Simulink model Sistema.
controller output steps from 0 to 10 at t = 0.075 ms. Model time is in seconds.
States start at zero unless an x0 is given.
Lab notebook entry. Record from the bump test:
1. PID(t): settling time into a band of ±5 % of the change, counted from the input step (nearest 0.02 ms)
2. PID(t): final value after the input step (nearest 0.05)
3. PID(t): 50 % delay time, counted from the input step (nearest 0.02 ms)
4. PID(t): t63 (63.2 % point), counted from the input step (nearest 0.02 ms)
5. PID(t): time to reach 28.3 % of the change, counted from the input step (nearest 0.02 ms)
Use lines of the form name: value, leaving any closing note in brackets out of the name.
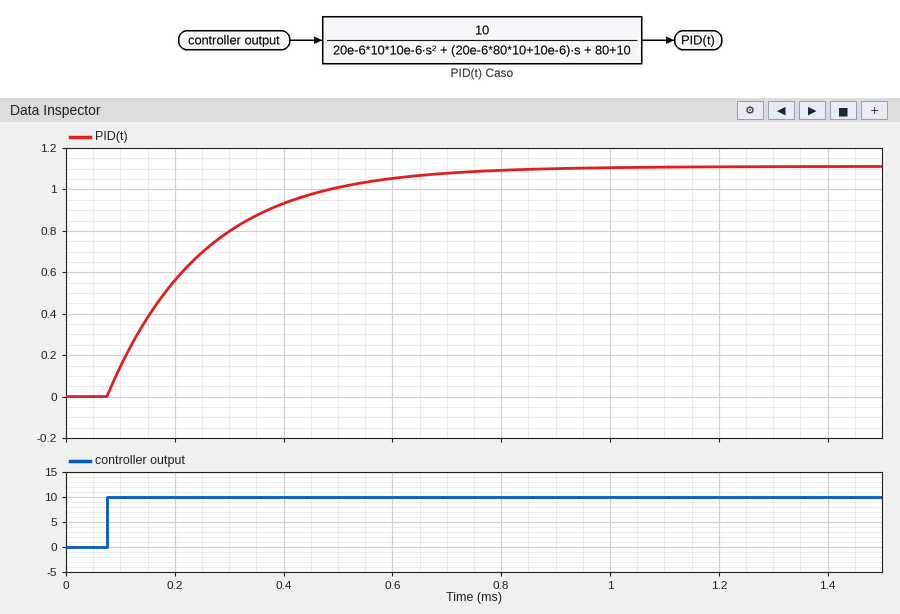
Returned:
PID(t): settling time into a band of ±5 % of the change, counted from the input step: 0.54 ms
PID(t): final value after the input step: 1.10
PID(t): 50 % delay time, counted from the input step: 0.12 ms
PID(t): t63 (63.2 % point), counted from the input step: 0.18 ms
PID(t): time to reach 28.3 % of the change, counted from the input step: 0.06 ms
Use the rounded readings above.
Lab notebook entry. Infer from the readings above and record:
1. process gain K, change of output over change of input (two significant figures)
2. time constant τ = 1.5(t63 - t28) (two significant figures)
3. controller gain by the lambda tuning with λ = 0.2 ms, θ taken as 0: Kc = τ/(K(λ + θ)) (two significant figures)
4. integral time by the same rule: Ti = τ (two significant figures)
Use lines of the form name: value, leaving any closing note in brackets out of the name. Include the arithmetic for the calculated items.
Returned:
process gain K, change of output over change of input: (1.1 - 0) / 10 = 0.11
time constant τ = 1.5(t63 - t28): 1.5 × (0.18 - 0.06) = 0.18 ms
controller gain by the lambda tuning with λ = 0.2 ms, θ taken as 0: Kc = τ/(K(λ + θ)): 0.18 / (0.11 × (0.2 + 0)) = 8.2
integral time by the same rule: Ti = τ: 0.18 ms
